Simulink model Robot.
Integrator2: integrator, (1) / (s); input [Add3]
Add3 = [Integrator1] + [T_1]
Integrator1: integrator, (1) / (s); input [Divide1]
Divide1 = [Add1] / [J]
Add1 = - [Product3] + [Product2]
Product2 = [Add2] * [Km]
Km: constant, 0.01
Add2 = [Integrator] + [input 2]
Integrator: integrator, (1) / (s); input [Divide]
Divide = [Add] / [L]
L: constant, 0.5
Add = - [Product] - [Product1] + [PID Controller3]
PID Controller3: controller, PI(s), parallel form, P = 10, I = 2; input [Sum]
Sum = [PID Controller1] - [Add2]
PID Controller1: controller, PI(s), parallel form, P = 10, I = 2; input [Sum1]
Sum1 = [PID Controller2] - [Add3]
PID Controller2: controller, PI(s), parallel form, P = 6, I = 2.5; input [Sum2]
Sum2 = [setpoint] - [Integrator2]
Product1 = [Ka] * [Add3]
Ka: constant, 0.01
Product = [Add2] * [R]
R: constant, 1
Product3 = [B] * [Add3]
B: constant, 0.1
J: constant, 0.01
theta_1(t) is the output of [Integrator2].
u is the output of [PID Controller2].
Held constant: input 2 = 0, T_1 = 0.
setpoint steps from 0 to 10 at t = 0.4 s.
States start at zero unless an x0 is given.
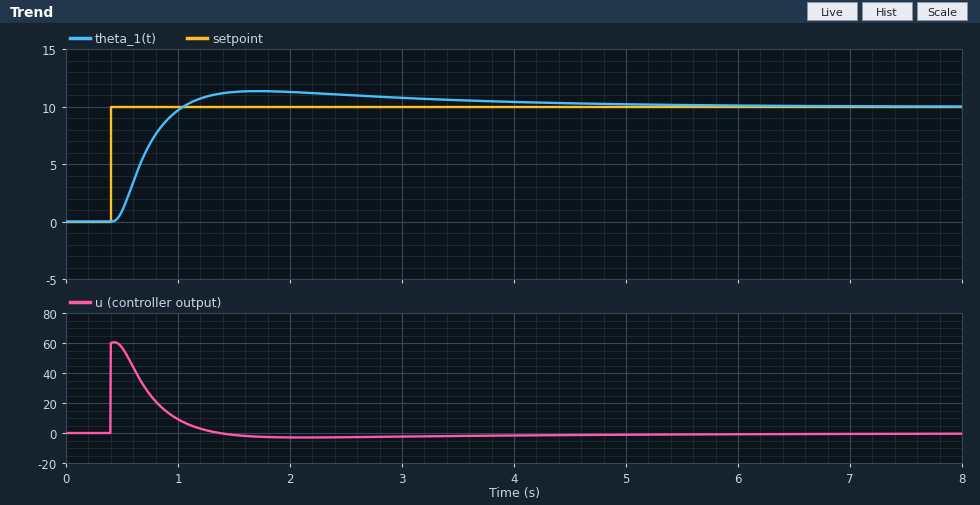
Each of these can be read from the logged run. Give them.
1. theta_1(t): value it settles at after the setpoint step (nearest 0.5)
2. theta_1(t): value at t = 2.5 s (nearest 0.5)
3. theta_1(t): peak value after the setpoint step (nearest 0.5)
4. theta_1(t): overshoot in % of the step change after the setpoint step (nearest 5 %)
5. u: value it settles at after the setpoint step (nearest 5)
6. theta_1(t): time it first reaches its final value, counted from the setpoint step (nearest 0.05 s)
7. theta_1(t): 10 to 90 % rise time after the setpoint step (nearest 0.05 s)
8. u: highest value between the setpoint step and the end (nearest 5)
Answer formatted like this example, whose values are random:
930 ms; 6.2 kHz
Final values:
10.0; 11.0; 11.5; 15 %; 0; 0.65 s; 0.40 s; 60
